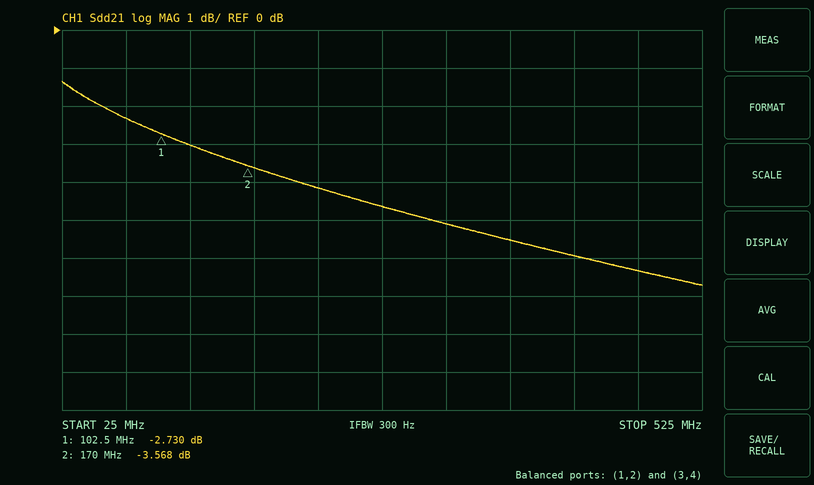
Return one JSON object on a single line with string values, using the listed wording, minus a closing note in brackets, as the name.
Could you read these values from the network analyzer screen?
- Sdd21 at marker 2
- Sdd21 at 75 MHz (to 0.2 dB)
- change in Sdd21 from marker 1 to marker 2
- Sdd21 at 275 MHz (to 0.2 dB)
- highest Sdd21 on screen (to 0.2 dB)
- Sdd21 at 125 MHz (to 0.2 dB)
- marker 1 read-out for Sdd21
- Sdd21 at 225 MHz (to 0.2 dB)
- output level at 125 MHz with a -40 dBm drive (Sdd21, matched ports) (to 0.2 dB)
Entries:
{"Sdd21 at marker 2": "-3.568 dB", "Sdd21 at 75 MHz": "-2.4 dB", "change in Sdd21 from marker 1 to marker 2": "-0.838 dB", "Sdd21 at 275 MHz": "-4.6 dB", "highest Sdd21 on screen": "-1.4 dB", "Sdd21 at 125 MHz": "-3.0 dB", "marker 1 read-out for Sdd21": "-2.730 dB", "Sdd21 at 225 MHz": "-4.2 dB", "output level at 125 MHz with a -40 dBm drive (Sdd21, matched ports)": "-43.0 dBm"}
